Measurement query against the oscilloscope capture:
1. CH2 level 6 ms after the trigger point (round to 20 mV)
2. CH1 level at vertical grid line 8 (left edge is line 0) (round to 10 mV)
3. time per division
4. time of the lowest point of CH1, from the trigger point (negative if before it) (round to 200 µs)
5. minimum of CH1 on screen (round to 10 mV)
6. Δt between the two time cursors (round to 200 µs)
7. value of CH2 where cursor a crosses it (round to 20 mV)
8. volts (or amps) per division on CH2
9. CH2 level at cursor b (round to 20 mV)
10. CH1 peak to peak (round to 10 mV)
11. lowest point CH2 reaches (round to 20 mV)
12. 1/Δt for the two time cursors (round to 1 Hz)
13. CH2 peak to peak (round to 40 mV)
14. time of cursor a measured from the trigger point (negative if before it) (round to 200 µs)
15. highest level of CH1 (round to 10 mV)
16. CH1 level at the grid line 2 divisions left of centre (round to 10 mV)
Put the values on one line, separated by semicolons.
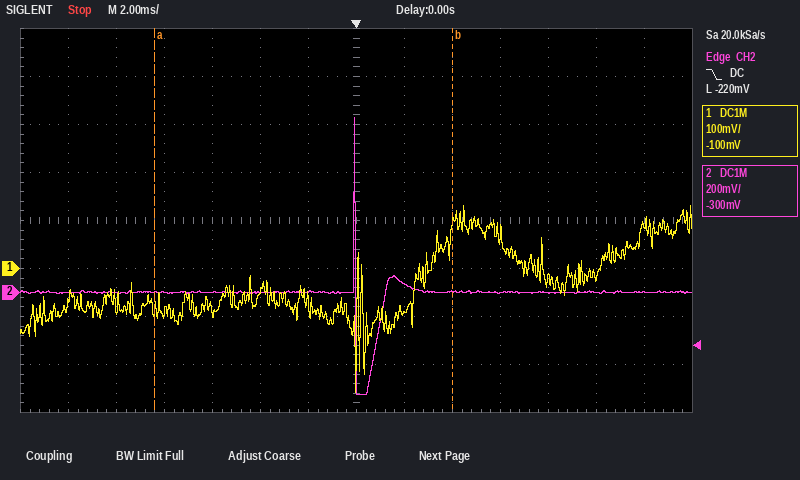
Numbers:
0 mV; -90 mV; 2 ms; 0.0 ms; -260 mV; 12.4 ms; 0 mV; 200 mV; 0 mV; 390 mV; -420 mV; 81 Hz; 1.16 V; -8.4 ms; 130 mV; -50 mV
